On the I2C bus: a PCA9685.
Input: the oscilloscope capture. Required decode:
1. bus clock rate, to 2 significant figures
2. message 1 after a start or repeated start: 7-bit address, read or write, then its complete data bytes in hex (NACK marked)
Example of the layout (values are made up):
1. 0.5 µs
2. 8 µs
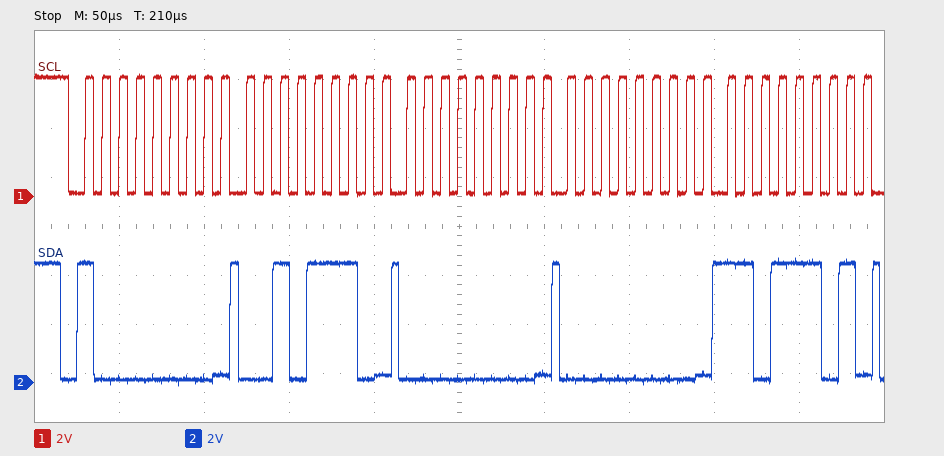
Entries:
1. 100 kHz
2. 0x40 write: 2E 00 00 DD
